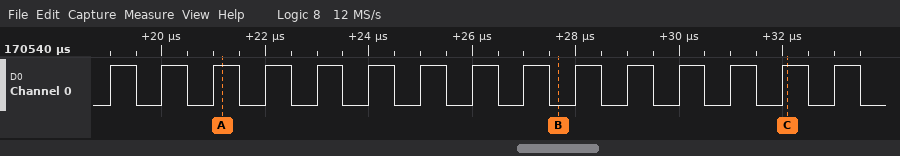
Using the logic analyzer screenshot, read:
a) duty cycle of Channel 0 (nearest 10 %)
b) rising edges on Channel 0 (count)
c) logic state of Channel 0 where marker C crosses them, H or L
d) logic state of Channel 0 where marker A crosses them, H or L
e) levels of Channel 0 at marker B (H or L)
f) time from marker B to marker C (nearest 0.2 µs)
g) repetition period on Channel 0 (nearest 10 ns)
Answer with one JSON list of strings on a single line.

["50 %", "15", "Channel 0=H", "Channel 0=H", "Channel 0=L", "4.4 µs", "1000 ns"]
